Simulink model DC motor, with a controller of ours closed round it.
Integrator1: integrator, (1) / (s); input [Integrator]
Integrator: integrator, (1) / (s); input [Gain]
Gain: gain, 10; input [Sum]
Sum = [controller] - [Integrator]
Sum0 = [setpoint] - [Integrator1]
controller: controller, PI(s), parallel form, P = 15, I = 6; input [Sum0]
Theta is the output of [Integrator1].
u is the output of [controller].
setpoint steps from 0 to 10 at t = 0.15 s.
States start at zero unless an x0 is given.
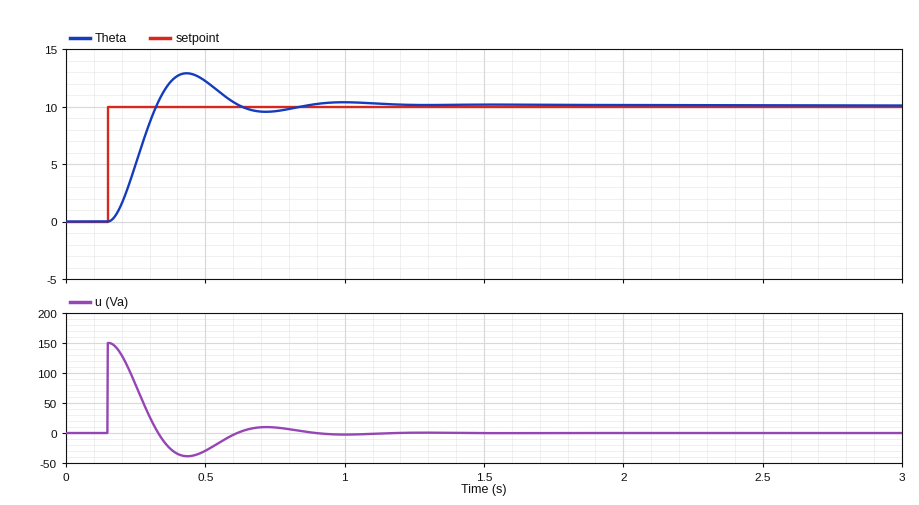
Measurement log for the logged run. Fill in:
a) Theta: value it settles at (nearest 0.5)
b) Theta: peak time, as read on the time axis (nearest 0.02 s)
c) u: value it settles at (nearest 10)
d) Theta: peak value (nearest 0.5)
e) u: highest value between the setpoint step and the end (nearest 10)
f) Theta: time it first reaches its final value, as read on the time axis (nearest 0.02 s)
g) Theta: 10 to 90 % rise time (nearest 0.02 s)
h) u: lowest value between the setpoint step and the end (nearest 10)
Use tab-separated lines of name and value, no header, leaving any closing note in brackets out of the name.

Theta: value it settles at	10.0
Theta: peak time, as read on the time axis	0.44 s
u: value it settles at	0
Theta: peak value	13.0
u: highest value between the setpoint step and the end	150
Theta: time it first reaches its final value, as read on the time axis	0.32 s
Theta: 10 to 90 % rise time	0.12 s
u: lowest value between the setpoint step and the end	-40
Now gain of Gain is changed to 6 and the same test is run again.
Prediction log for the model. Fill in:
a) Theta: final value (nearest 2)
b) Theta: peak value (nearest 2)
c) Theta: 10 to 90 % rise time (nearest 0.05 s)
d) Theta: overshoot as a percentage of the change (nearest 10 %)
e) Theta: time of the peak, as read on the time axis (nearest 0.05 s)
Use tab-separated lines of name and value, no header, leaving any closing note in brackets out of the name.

Theta: final value	10
Theta: peak value	14
Theta: 10 to 90 % rise time	0.15 s
Theta: overshoot as a percentage of the change	40 %
Theta: time of the peak, as read on the time axis	0.50 s
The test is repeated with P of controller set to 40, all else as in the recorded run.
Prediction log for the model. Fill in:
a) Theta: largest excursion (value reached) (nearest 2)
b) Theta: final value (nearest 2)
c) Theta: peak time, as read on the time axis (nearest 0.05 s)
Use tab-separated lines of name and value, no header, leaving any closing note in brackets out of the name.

Theta: largest excursion (value reached)	14
Theta: final value	10
Theta: peak time, as read on the time axis	0.30 s
